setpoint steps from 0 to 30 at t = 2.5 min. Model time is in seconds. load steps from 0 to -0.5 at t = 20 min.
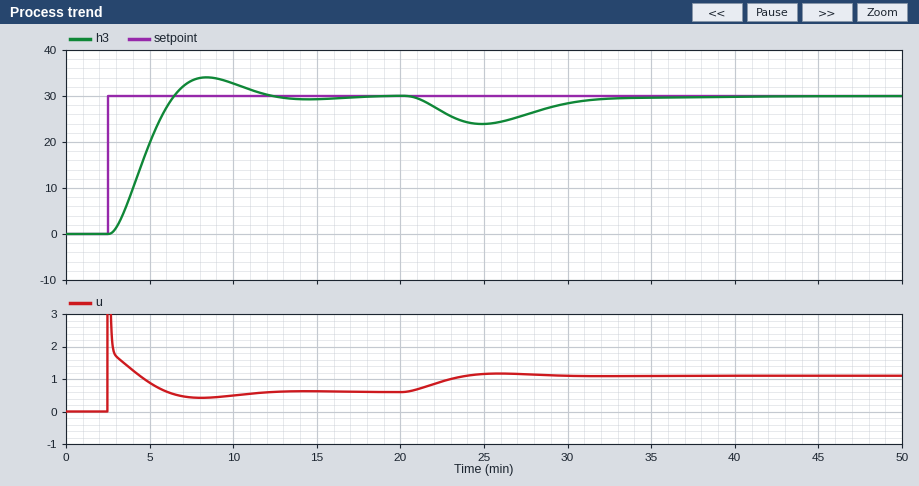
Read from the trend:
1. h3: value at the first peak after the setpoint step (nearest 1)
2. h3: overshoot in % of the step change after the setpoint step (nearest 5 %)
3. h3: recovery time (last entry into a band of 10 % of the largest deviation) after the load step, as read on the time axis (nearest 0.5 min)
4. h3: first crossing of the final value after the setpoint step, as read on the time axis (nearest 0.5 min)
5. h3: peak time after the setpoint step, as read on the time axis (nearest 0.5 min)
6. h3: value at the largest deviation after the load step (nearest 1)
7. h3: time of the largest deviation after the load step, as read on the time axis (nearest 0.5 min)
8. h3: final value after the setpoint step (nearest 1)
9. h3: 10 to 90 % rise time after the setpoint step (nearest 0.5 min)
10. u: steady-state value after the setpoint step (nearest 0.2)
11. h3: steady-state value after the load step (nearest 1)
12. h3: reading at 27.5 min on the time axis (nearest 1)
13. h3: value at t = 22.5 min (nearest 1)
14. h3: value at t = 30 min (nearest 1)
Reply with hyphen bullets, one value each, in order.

- 34
- 15 %
- 32.5 min
- 6.5 min
- 8.5 min
- 24
- 25.0 min
- 30
- 2.5 min
- 0.6
- 30
- 26
- 27
- 28
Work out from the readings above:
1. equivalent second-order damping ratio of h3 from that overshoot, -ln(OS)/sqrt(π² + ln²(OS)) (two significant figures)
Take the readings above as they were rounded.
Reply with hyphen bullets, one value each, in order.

- 0.52
